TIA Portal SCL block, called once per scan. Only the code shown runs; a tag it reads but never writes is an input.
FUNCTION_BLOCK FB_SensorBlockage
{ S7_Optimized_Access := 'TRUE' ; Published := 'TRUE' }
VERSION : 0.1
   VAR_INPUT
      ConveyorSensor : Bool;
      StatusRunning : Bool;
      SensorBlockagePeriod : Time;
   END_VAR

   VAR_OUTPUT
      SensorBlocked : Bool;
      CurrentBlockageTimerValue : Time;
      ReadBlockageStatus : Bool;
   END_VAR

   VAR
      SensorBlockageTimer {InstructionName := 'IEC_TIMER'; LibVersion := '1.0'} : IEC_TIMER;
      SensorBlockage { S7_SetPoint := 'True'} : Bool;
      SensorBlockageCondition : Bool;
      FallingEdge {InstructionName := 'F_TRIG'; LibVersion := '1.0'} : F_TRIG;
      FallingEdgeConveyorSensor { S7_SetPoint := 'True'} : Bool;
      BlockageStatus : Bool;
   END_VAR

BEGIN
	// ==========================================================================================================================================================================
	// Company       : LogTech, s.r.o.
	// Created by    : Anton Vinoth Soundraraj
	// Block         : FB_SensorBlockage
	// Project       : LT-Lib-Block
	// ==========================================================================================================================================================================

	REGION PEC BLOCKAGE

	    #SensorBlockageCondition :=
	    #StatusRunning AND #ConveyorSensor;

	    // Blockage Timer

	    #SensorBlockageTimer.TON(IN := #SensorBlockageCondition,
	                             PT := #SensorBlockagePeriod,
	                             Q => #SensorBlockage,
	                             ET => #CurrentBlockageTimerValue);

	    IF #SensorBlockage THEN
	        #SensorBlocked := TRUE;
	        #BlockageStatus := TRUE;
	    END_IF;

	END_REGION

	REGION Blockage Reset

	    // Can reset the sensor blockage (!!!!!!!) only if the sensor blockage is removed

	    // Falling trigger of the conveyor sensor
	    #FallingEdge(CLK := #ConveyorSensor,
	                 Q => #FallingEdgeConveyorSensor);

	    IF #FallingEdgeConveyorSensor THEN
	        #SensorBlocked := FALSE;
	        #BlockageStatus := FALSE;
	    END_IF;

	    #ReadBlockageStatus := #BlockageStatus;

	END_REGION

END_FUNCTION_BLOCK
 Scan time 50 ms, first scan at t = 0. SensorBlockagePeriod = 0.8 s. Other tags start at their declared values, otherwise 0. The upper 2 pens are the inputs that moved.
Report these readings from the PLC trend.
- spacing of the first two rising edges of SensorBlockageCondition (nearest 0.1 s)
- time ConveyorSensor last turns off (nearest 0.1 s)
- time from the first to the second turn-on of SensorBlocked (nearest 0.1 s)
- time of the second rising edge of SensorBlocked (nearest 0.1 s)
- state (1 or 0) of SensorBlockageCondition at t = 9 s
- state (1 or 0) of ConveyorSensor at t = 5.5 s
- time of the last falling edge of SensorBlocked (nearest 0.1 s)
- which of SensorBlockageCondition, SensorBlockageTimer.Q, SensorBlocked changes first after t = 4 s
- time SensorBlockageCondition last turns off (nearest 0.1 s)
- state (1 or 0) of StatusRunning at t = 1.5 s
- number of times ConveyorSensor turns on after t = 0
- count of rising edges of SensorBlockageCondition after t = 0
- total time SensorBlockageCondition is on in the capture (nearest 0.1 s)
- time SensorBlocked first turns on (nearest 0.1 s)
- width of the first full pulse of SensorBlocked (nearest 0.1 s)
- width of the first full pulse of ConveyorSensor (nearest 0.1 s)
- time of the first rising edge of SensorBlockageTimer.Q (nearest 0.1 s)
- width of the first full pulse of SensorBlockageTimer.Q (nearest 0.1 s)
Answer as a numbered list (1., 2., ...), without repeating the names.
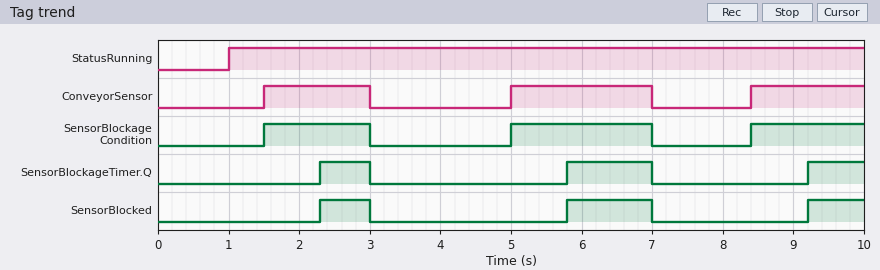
1. 3.5 s
2. 7.0 s
3. 3.5 s
4. 5.8 s
5. 1
6. 1
7. 7.0 s
8. SensorBlockageCondition
9. 7.0 s
10. 1
11. 3
12. 3
13. 5.1 s
14. 2.3 s
15. 0.7 s
16. 1.5 s
17. 2.3 s
18. 0.7 s
